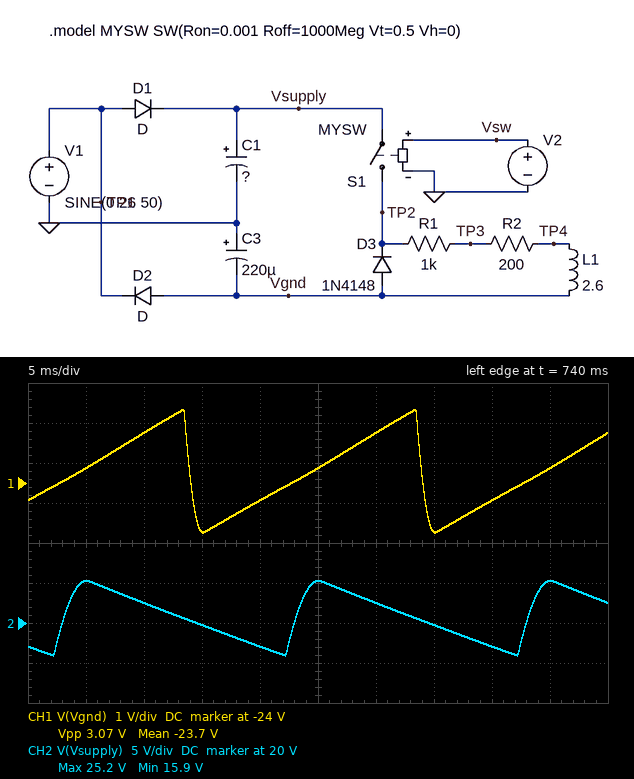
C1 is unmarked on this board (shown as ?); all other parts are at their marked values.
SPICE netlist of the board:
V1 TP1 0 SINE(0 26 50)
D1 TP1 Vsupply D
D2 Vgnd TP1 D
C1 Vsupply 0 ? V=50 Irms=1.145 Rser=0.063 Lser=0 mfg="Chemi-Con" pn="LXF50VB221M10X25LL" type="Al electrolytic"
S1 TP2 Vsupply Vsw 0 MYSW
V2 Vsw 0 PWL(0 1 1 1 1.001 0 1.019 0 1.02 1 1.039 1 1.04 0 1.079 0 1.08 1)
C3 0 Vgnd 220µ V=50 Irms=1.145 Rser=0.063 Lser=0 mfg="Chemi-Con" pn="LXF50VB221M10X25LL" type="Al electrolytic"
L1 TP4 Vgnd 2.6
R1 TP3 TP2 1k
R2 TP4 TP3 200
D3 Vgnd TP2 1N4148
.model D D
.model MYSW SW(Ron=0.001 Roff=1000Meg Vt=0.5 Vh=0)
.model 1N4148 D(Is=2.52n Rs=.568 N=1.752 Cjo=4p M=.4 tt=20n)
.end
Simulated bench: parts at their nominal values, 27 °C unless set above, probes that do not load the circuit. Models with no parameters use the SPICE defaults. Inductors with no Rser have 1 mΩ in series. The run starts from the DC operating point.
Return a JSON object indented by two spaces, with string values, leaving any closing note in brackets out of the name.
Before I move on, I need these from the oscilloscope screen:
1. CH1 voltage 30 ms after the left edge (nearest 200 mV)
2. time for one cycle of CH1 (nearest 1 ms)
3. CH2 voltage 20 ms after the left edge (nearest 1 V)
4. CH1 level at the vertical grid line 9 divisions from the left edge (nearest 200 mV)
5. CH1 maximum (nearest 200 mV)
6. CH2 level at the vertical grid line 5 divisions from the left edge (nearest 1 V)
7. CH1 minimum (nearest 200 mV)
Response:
{
  "CH1 voltage 30 ms after the left edge": "-22.8 V",
  "time for one cycle of CH1": "20 ms",
  "CH2 voltage 20 ms after the left edge": "17 V",
  "CH1 level at the vertical grid line 9 divisions from the left edge": "-23.6 V",
  "CH1 maximum": "-22.2 V",
  "CH2 level at the vertical grid line 5 divisions from the left edge": "25 V",
  "CH1 minimum": "-25.2 V"
}
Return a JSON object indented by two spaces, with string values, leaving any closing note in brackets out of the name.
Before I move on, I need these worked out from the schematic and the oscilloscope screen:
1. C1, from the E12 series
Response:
{
  "C1, from the E12 series": "68 µF"
}
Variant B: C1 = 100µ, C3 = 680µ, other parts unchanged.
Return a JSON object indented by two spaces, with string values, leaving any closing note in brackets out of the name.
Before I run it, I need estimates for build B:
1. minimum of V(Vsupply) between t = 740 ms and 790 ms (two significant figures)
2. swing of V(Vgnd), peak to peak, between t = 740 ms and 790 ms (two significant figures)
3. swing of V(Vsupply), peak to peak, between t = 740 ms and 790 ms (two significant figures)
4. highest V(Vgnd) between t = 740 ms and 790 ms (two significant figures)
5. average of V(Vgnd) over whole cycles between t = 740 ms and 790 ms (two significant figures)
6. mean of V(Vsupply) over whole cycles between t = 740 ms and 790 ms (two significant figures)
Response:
{
  "minimum of V(Vsupply) between t = 740 ms and 790 ms": "18 V",
  "swing of V(Vgnd), peak to peak, between t = 740 ms and 790 ms": "1.1 V",
  "swing of V(Vsupply), peak to peak, between t = 740 ms and 790 ms": "6.8 V",
  "highest V(Vgnd) between t = 740 ms and 790 ms": "-24 V",
  "average of V(Vgnd) over whole cycles between t = 740 ms and 790 ms": "-25 V",
  "mean of V(Vsupply) over whole cycles between t = 740 ms and 790 ms": "22 V"
}
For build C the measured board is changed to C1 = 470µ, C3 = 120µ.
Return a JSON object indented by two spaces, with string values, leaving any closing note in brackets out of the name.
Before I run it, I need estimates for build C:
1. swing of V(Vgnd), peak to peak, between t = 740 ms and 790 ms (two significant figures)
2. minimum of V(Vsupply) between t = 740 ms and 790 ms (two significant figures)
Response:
{
  "swing of V(Vgnd), peak to peak, between t = 740 ms and 790 ms": "5.8 V",
  "minimum of V(Vsupply) between t = 740 ms and 790 ms": "24 V"
}
